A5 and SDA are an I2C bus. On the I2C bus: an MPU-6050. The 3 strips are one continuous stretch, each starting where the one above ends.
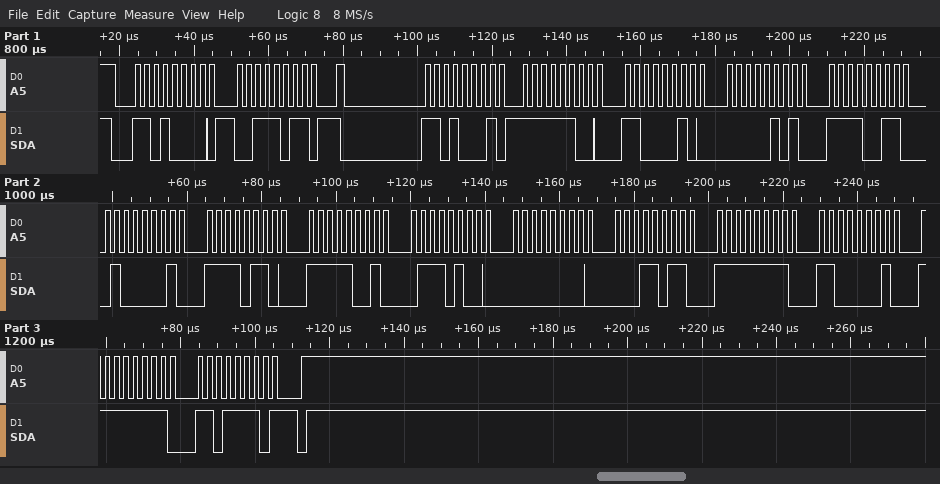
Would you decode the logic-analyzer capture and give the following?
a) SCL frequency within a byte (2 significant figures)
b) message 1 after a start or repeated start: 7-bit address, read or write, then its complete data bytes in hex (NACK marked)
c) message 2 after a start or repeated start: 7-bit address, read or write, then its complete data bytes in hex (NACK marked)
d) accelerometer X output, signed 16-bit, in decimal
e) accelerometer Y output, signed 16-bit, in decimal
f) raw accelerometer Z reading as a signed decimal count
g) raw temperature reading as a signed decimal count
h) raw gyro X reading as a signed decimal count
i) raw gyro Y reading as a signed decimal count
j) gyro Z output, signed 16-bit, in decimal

400 kHz
0x68 write: 3B
0x68 read: FC C2 05 F3 41 F6 F9 74 00 1B FF C1 FF DE NACK
-830
1523
16886
-1676
27
-63
-34
